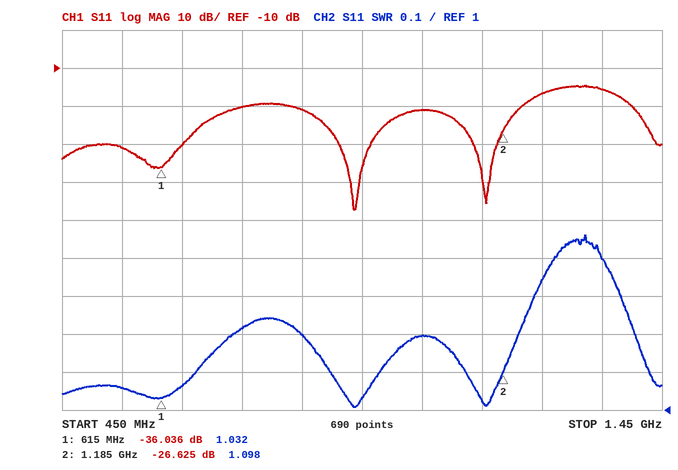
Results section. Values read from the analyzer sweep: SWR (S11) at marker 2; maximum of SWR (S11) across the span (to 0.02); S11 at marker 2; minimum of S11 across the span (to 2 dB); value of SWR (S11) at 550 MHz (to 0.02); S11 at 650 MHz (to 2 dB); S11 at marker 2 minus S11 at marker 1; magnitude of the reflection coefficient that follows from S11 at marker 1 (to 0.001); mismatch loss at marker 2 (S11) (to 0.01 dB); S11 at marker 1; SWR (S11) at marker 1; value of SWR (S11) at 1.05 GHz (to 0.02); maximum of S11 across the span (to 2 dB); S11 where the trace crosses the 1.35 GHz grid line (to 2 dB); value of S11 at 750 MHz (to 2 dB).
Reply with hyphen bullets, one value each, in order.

- 1.098
- 1.46
- -26.625 dB
- -48 dB
- 1.06
- -30 dB
- 9.411 dB
- 0.016
- 0.01 dB
- -36.036 dB
- 1.032
- 1.20
- -14 dB
- -16 dB
- -20 dB
